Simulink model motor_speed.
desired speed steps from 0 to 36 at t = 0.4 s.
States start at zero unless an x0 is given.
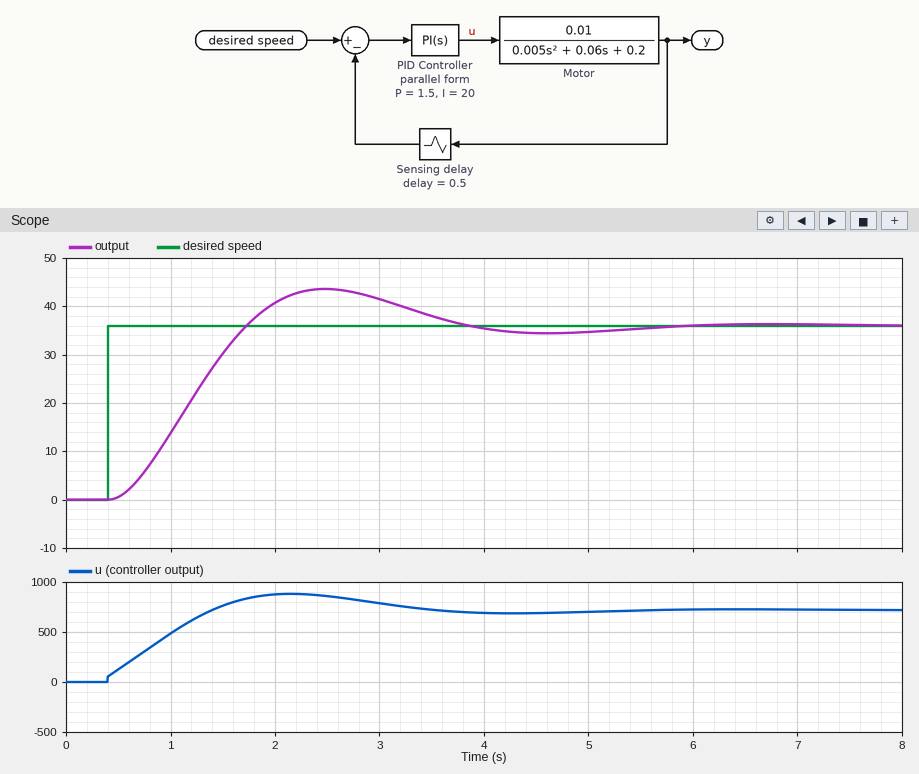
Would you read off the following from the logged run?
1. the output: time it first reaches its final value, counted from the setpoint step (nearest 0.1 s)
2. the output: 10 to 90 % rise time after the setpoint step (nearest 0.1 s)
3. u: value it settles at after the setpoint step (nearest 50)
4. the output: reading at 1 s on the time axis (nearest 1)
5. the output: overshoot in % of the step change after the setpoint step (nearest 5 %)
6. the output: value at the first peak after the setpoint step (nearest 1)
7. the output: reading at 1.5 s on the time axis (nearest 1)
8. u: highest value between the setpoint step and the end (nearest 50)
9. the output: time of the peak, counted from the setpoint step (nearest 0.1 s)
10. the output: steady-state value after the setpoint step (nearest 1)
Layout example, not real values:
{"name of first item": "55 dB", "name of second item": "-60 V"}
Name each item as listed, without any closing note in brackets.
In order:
{"the output: time it first reaches its final value, counted from the setpoint step": "1.3 s", "the output: 10 to 90 % rise time after the setpoint step": "0.9 s", "u: value it settles at after the setpoint step": "700", "the output: reading at 1 s on the time axis": "14", "the output: overshoot in % of the step change after the setpoint step": "20 %", "the output: value at the first peak after the setpoint step": "44", "the output: reading at 1.5 s on the time axis": "30", "u: highest value between the setpoint step and the end": "900", "the output: time of the peak, counted from the setpoint step": "2.1 s", "the output: steady-state value after the setpoint step": "36"}
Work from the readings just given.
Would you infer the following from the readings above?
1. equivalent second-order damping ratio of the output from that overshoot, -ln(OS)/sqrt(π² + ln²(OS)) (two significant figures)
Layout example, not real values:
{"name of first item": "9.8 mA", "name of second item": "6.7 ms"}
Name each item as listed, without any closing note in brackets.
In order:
{"equivalent second-order damping ratio of the output from that overshoot, -ln(OS)/sqrt(π² + ln²(OS))": "0.46"}
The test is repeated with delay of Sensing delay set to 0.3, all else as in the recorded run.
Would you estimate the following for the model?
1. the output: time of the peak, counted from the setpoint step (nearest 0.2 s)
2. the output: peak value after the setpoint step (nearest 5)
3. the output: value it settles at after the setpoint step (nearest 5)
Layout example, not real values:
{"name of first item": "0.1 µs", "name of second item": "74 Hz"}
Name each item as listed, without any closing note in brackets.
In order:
{"the output: time of the peak, counted from the setpoint step": "2.2 s", "the output: peak value after the setpoint step": "40", "the output: value it settles at after the setpoint step": "35"}
